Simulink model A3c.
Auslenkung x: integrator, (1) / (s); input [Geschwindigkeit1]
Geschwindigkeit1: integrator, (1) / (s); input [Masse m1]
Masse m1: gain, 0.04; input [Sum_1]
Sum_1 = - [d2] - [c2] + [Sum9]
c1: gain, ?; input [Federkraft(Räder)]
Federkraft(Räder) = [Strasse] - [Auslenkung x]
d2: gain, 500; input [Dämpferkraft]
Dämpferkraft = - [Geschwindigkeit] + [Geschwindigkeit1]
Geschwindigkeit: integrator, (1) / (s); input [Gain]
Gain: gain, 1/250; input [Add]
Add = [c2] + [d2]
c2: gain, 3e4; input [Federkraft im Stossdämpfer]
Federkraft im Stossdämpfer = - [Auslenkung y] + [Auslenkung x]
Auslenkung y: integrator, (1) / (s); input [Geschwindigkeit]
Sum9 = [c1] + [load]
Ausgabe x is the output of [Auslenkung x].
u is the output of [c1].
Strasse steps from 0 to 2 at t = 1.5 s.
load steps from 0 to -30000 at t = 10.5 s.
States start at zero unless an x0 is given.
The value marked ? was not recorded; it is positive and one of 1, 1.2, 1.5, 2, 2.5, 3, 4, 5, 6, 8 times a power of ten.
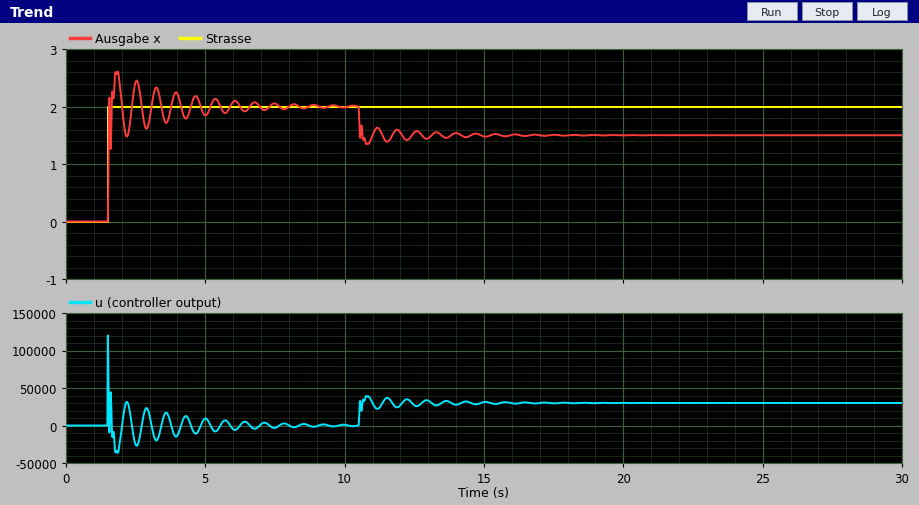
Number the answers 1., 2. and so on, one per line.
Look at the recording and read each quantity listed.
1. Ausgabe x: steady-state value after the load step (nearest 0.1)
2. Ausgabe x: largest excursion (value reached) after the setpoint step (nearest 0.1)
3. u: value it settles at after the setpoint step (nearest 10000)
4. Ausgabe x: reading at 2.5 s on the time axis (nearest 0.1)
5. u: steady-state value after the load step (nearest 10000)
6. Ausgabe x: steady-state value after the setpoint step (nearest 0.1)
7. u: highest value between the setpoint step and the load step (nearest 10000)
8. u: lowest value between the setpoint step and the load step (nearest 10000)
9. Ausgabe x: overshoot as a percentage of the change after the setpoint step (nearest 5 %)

1. 1.5
2. 2.6
3. 0
4. 2.4
5. 30000
6. 2.0
7. 120000
8. -40000
9. 30 %
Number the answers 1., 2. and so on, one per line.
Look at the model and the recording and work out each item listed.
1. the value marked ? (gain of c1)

1. 60000
